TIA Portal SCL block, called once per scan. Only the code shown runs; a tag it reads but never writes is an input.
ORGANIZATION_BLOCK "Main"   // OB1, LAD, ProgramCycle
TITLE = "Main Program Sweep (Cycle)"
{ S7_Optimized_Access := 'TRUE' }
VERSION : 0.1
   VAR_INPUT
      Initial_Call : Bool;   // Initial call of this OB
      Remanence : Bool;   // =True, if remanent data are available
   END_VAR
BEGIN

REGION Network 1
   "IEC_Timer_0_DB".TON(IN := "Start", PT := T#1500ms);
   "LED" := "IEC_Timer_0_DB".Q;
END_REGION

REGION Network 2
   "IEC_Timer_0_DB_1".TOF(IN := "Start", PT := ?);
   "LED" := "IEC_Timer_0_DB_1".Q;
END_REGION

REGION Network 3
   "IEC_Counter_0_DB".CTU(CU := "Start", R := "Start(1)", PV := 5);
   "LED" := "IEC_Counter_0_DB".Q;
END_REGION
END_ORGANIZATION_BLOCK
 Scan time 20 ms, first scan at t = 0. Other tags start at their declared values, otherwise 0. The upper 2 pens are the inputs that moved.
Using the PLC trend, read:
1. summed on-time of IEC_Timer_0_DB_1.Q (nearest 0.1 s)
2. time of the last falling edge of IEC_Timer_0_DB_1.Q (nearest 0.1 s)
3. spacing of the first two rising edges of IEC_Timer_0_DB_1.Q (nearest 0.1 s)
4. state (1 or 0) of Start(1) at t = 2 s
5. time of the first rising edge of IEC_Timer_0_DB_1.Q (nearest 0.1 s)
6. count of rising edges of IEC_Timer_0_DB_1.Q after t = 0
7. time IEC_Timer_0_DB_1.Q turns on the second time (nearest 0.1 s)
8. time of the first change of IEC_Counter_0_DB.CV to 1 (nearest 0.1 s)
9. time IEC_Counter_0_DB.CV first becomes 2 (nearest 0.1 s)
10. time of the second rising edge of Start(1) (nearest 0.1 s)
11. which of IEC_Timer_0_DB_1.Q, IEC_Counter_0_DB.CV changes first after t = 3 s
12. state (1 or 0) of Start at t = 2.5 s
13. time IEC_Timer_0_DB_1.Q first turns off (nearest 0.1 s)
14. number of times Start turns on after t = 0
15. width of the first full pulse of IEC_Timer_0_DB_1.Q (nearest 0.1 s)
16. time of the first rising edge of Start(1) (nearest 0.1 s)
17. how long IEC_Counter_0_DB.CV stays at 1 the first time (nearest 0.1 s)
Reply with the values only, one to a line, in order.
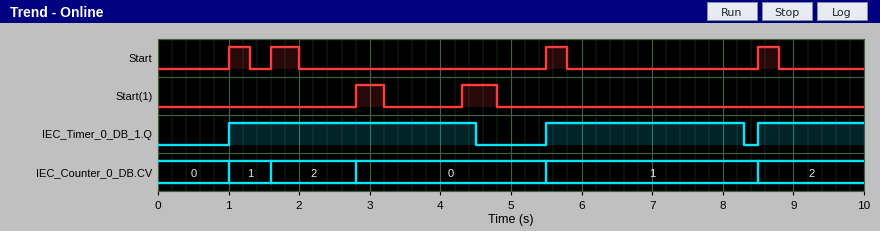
7.8 s
8.3 s
4.5 s
0
1.0 s
3
5.5 s
1.0 s
1.6 s
4.3 s
IEC_Timer_0_DB_1.Q
0
4.5 s
4
3.5 s
2.8 s
0.6 s
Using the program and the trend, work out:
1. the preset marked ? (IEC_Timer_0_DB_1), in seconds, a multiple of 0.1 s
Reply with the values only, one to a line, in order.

2.5 s
